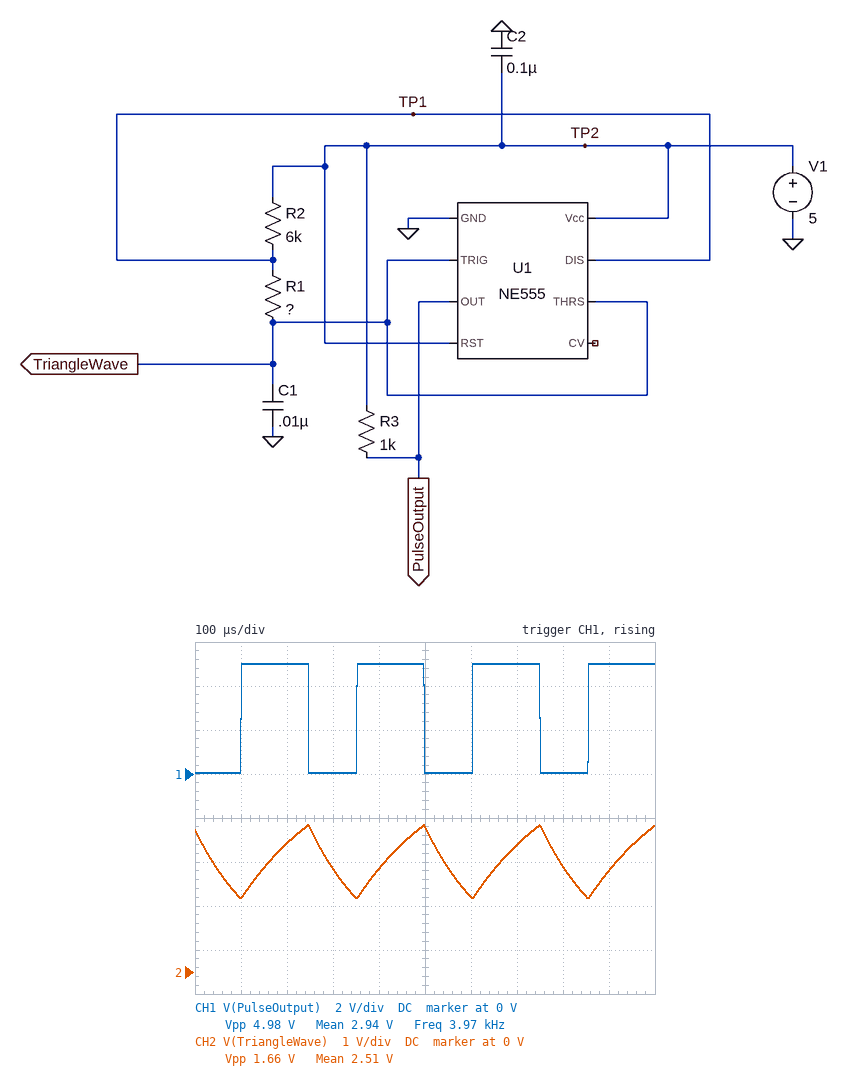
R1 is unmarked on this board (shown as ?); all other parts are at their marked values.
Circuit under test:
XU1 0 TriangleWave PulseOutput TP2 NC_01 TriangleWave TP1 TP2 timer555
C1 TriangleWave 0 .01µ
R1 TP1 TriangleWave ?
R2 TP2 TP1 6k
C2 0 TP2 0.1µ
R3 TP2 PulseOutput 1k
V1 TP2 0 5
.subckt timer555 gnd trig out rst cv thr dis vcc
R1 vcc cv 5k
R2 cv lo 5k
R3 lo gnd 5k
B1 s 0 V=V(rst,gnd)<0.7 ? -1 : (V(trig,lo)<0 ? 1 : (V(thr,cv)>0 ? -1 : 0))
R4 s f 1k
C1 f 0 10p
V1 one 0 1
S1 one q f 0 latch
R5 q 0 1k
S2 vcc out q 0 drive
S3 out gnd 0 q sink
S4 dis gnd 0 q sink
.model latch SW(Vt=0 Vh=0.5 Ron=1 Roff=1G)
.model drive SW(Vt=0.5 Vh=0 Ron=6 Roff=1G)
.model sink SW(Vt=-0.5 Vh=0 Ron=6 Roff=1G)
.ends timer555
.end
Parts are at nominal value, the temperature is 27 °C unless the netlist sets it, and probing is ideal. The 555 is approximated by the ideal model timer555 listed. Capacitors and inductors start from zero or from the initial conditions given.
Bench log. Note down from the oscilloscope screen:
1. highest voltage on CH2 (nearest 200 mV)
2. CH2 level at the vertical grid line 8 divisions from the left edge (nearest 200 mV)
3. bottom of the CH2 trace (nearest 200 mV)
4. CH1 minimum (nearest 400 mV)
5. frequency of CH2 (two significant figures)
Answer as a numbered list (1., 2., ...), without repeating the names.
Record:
1. 3.4 V
2. 2.4 V
3. 1.6 V
4. 0 V
5. 4.0 kHz
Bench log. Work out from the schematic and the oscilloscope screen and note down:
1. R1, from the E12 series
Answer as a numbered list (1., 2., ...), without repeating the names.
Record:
1. 15 kΩ
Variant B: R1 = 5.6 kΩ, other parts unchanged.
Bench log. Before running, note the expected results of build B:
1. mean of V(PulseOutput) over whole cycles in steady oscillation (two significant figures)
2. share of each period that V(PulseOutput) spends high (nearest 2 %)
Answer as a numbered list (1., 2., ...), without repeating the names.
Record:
1. 3.4 V
2. 68 %
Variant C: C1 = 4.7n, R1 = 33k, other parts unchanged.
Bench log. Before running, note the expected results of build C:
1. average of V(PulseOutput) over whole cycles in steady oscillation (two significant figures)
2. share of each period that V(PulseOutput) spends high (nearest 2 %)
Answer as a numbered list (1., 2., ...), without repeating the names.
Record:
1. 2.7 V
2. 54 %
